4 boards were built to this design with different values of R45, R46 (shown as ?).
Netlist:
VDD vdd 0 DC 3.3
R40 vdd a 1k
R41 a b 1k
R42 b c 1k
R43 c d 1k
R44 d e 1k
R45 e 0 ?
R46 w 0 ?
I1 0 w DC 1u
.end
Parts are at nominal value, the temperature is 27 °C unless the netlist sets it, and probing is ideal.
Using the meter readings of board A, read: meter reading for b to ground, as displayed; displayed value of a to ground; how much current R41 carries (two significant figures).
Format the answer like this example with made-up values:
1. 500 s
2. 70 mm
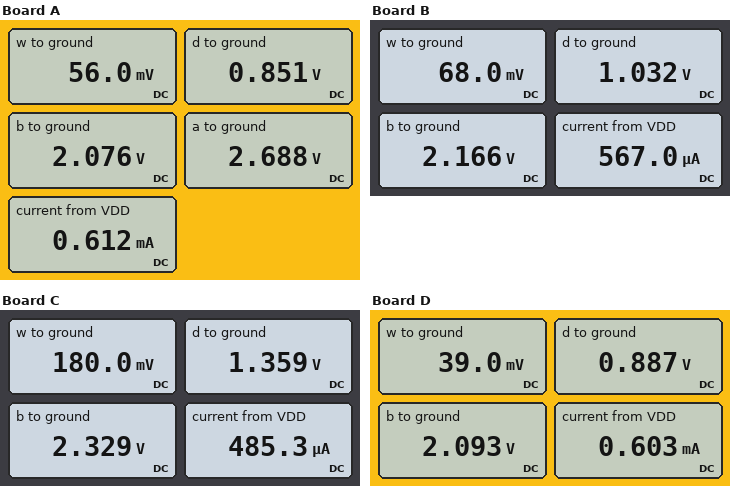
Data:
1. 2.076 V
2. 2.688 V
3. 610 µA
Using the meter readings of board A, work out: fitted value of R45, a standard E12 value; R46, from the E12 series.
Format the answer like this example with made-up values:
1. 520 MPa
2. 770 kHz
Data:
1. 390 Ω
2. 56 kΩ
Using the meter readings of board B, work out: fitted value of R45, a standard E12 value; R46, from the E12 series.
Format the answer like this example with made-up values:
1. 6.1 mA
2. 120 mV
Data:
1. 820 Ω
2. 68 kΩ
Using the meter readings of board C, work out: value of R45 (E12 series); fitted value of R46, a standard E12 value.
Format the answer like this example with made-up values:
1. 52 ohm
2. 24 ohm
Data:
1. 1.8 kΩ
2. 180 kΩ
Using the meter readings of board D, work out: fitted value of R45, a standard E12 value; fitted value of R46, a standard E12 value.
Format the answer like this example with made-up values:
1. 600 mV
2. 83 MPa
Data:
1. 470 Ω
2. 39 kΩ
